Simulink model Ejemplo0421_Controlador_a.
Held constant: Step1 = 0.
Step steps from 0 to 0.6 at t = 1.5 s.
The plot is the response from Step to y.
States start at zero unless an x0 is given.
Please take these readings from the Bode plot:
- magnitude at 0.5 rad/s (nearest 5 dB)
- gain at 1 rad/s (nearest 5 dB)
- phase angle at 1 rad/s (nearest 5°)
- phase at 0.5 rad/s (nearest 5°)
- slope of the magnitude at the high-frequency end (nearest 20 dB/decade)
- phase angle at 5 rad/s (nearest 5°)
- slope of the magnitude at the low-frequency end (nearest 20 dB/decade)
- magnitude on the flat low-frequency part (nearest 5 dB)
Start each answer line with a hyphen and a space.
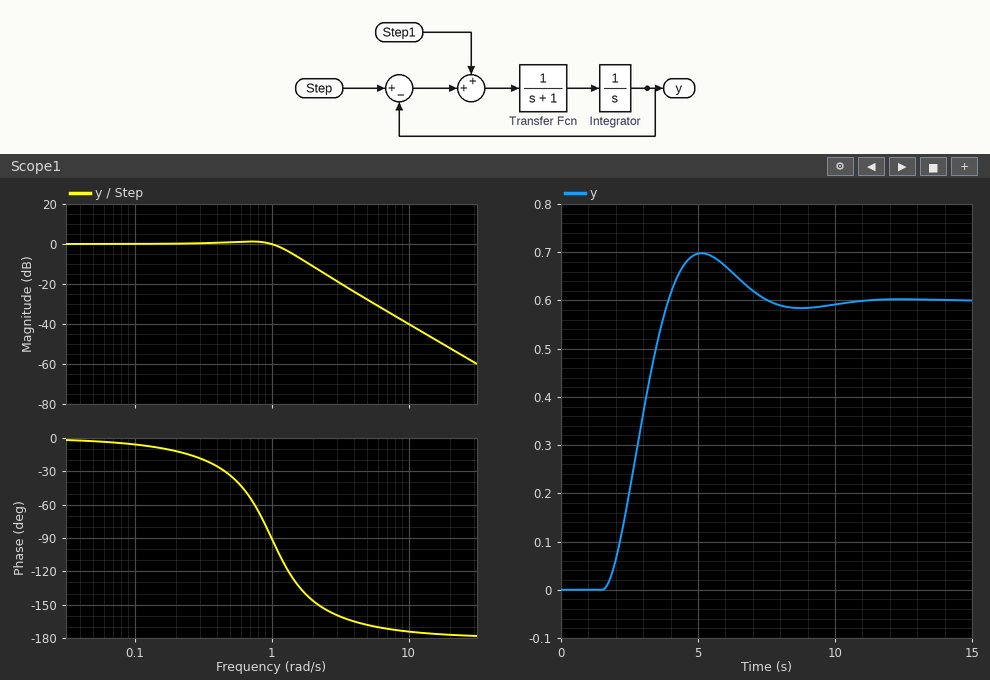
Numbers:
- 0 dB
- 0 dB
- -90°
- -35°
- -40 dB/decade
- -170°
- 0 dB/decade
- 0 dB
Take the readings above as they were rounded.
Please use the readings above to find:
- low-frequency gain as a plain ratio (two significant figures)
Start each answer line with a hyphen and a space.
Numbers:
- 1.0
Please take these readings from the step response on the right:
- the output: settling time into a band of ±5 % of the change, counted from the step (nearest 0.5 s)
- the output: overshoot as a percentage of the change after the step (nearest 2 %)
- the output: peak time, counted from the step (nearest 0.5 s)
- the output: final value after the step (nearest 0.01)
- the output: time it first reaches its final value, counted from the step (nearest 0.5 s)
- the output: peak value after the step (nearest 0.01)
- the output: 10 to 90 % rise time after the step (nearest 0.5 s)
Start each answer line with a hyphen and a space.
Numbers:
- 5.5 s
- 16 %
- 3.5 s
- 0.60
- 2.5 s
- 0.70
- 1.5 s
